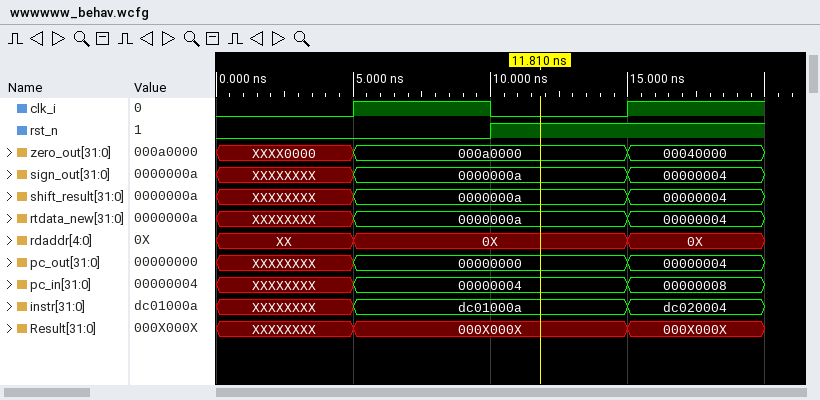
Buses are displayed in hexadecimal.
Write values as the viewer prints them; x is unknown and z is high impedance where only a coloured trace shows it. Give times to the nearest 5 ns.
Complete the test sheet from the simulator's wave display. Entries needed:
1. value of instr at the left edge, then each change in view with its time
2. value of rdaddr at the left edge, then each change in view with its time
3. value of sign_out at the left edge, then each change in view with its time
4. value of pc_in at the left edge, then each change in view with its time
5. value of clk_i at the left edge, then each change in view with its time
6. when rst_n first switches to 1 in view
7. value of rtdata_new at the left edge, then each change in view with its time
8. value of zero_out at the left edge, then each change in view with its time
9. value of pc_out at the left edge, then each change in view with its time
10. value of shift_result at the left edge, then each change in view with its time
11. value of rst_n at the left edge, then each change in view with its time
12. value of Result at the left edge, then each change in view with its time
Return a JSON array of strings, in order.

["XXXXXXXX, dc01000a at 5 ns, dc020004 at 15 ns", "XX, 0X at 5 ns, 0X at 15 ns", "XXXXXXXX, 0000000a at 5 ns, 00000004 at 15 ns", "XXXXXXXX, 00000004 at 5 ns, 00000008 at 15 ns", "0, 1 at 5 ns, 0 at 10 ns, 1 at 15 ns", "10 ns", "XXXXXXXX, 0000000a at 5 ns, 00000004 at 15 ns", "XXXX0000, 000a0000 at 5 ns, 00040000 at 15 ns", "XXXXXXXX, 00000000 at 5 ns, 00000004 at 15 ns", "XXXXXXXX, 0000000a at 5 ns, 00000004 at 15 ns", "0, 1 at 10 ns", "XXXXXXXX, 000X000X at 5 ns, 000X000X at 15 ns"]
